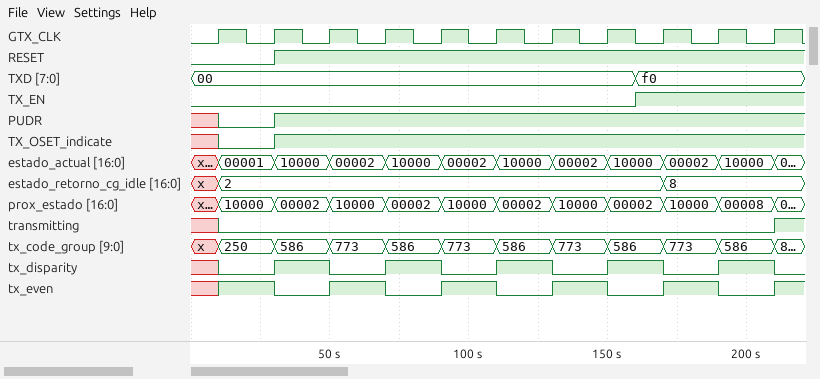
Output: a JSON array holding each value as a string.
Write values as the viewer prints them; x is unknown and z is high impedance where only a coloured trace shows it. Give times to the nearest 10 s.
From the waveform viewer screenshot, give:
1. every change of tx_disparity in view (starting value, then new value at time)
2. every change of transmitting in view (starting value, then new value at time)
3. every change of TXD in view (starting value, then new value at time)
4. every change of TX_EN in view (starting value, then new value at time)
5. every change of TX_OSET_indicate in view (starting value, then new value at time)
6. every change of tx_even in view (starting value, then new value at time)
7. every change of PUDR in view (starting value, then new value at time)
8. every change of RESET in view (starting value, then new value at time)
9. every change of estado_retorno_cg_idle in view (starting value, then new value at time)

["x, 0 at 10 s, 1 at 30 s, 0 at 50 s, 1 at 70 s, 0 at 90 s, 1 at 110 s, 0 at 130 s, 1 at 150 s, 0 at 170 s, 1 at 190 s, 0 at 210 s", "x, 0 at 10 s, 1 at 210 s", "00, f0 at 160 s", "0, 1 at 160 s", "x, 0 at 10 s, 1 at 30 s", "x, 1 at 10 s, 0 at 30 s, 1 at 50 s, 0 at 70 s, 1 at 90 s, 0 at 110 s, 1 at 130 s, 0 at 150 s, 1 at 170 s, 0 at 190 s, 1 at 210 s", "x, 0 at 10 s, 1 at 30 s", "0, 1 at 30 s", "x, 2 at 10 s, 8 at 170 s"]
